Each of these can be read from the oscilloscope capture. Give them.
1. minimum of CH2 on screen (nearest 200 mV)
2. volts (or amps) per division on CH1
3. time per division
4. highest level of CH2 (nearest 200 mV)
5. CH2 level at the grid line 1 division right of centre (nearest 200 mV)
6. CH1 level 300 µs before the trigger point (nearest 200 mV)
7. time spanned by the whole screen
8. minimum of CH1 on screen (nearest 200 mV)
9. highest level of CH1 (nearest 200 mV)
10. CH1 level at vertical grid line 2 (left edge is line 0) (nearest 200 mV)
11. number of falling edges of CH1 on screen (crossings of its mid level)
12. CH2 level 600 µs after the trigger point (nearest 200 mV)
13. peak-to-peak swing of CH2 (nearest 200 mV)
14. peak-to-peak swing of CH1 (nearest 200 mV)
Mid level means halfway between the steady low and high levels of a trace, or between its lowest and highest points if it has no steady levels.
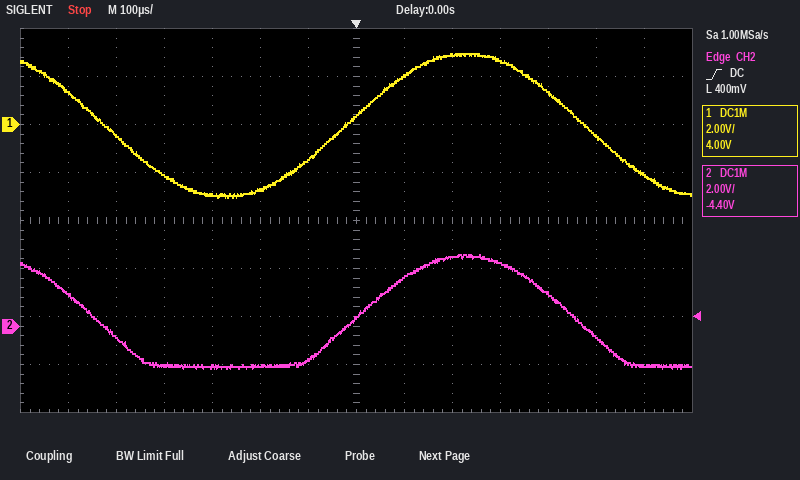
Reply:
-1.8 V
2 V
100 µs
3.0 V
2.0 V
-3.0 V
1.4 ms
-3.0 V
3.0 V
-400 mV
2
-1.6 V
4.8 V
6.0 V
